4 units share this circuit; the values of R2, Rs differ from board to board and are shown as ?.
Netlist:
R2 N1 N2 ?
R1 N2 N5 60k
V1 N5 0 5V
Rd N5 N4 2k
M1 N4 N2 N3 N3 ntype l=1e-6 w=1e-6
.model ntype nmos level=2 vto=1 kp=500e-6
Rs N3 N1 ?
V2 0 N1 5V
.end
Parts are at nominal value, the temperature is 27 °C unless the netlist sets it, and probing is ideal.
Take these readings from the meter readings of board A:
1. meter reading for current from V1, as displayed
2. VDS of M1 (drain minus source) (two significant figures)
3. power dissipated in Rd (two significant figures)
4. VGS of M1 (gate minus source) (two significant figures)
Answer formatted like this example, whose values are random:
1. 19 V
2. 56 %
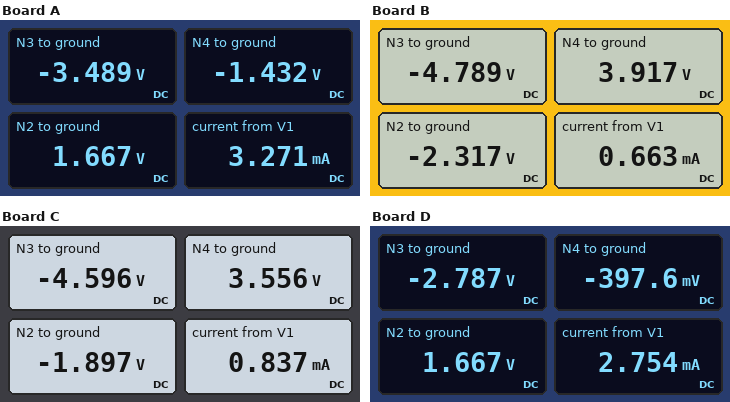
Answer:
1. 3.271 mA
2. 2.1 V
3. 21 mW
4. 5.2 V
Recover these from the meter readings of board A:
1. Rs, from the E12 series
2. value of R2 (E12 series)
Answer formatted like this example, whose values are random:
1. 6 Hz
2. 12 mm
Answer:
1. 470 Ω
2. 120 kΩ
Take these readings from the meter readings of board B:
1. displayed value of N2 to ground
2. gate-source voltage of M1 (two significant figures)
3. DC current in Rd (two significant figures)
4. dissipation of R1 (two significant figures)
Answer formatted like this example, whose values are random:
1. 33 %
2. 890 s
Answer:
1. -2.317 V
2. 2.5 V
3. 540 µA
4. 890 µW
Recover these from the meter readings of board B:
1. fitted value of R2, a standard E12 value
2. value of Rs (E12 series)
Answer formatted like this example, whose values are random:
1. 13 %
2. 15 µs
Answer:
1. 22 kΩ
2. 390 Ω
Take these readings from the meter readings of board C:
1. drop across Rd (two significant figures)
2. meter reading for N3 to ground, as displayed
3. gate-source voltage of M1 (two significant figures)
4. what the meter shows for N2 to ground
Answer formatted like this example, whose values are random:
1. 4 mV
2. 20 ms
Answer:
1. 1.4 V
2. -4.596 V
3. 2.7 V
4. -1.897 V
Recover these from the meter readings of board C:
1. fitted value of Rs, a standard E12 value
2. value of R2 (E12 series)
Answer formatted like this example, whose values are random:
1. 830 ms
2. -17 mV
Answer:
1. 560 Ω
2. 27 kΩ
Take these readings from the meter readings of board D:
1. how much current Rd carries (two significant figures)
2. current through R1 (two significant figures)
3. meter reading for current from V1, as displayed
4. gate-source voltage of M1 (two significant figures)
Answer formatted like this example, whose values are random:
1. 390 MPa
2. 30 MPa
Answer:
1. 2.7 mA
2. 56 µA
3. 2.754 mA
4. 4.5 V
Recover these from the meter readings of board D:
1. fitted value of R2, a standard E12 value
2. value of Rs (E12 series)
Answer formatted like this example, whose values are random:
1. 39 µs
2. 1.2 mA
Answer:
1. 120 kΩ
2. 820 Ω
